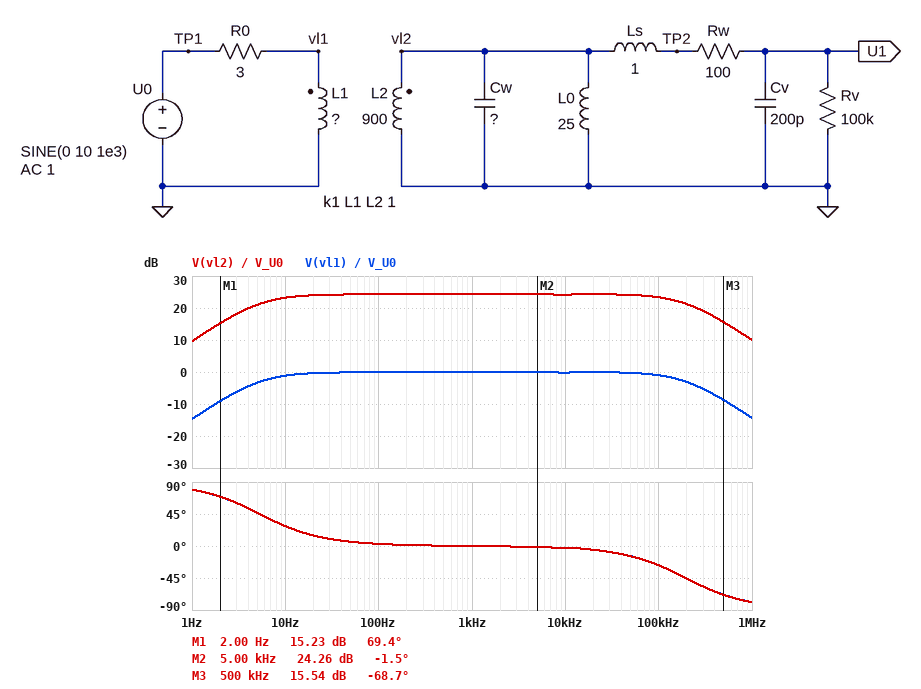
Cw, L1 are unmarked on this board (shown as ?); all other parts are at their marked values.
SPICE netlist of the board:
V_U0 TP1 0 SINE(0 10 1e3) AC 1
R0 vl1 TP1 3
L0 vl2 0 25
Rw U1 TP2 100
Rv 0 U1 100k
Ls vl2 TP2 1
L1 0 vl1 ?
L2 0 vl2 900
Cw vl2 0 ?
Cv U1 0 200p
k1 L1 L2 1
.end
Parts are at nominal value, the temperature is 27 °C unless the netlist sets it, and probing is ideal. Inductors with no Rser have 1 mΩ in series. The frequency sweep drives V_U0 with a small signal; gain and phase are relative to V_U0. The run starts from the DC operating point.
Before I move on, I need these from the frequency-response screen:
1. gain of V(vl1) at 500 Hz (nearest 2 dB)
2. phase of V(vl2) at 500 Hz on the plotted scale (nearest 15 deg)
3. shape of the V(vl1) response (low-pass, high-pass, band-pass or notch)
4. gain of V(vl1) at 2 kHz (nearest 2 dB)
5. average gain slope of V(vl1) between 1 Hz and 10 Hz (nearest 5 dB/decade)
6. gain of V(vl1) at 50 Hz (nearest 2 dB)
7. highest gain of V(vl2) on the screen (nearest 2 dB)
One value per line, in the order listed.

0 dB
0 deg
band-pass
0 dB
15 dB/decade
0 dB
24 dB
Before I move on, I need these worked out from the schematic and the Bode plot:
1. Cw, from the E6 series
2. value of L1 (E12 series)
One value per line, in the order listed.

1 nF
3.3 H
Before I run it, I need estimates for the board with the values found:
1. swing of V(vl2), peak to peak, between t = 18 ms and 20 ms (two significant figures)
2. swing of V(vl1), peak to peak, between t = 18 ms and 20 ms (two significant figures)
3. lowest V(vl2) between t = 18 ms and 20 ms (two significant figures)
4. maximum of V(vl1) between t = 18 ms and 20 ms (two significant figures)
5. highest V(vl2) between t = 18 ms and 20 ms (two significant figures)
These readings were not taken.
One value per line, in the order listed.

330 V
20 V
-160 V
9.9 V
160 V
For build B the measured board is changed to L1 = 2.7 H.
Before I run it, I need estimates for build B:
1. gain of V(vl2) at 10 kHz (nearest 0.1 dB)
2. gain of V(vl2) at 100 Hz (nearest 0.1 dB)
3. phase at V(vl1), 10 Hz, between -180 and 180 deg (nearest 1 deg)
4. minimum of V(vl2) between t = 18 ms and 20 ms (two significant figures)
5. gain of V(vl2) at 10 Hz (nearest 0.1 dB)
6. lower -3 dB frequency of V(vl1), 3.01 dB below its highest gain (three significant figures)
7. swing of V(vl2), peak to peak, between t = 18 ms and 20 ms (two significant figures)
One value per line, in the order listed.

25.0 dB
25.1 dB
33 deg
-180 V
23.6 dB
6.51 Hz
360 V
